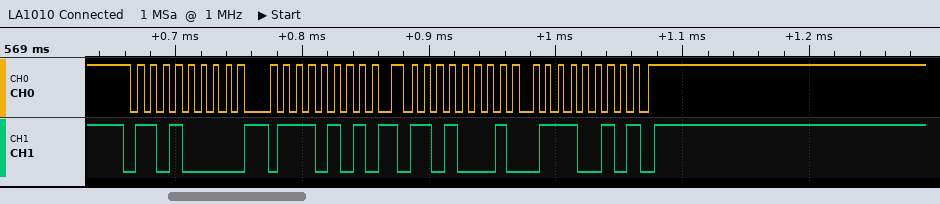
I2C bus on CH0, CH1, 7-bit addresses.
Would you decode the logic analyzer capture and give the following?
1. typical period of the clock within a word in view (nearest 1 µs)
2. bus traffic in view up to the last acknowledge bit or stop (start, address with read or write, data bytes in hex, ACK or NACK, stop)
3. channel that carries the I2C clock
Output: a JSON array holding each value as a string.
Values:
["10 µs", "start, address 68 write ACK, 75 ACK, repeated start, address 68 read ACK, 72 NACK, stop", "CH0"]
